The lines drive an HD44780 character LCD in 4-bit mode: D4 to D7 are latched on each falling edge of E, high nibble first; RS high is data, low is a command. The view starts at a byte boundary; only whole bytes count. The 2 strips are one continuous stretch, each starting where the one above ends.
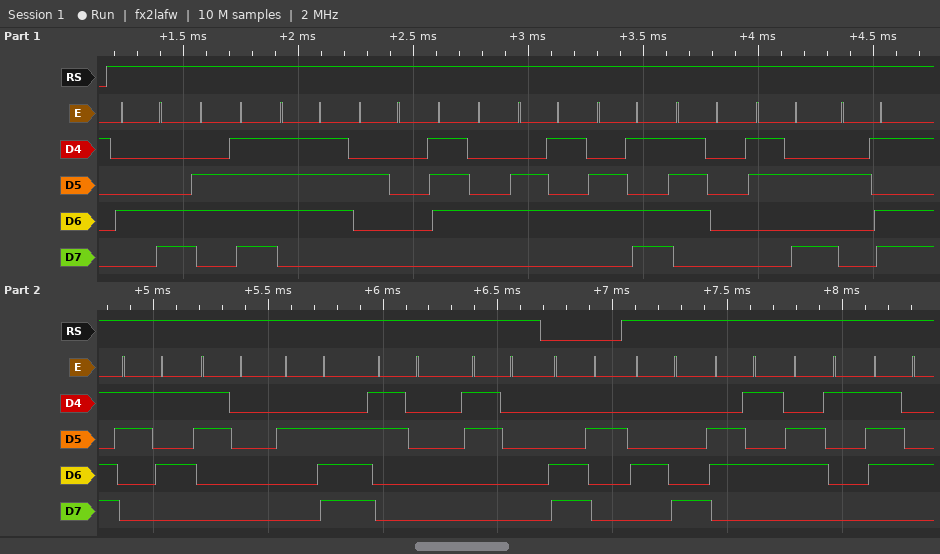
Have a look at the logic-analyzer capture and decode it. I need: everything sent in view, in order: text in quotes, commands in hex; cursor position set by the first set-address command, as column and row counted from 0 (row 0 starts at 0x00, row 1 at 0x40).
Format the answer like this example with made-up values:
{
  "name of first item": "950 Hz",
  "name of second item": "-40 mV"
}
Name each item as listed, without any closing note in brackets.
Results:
{
  "everything sent in view, in order: text in quotes, commands in hex": "\"Low temp:-50.00\" 0xC2 \"Heat\"",
  "cursor position set by the first set-address command, as column and row counted from 0": "column 2, row 1"
}
